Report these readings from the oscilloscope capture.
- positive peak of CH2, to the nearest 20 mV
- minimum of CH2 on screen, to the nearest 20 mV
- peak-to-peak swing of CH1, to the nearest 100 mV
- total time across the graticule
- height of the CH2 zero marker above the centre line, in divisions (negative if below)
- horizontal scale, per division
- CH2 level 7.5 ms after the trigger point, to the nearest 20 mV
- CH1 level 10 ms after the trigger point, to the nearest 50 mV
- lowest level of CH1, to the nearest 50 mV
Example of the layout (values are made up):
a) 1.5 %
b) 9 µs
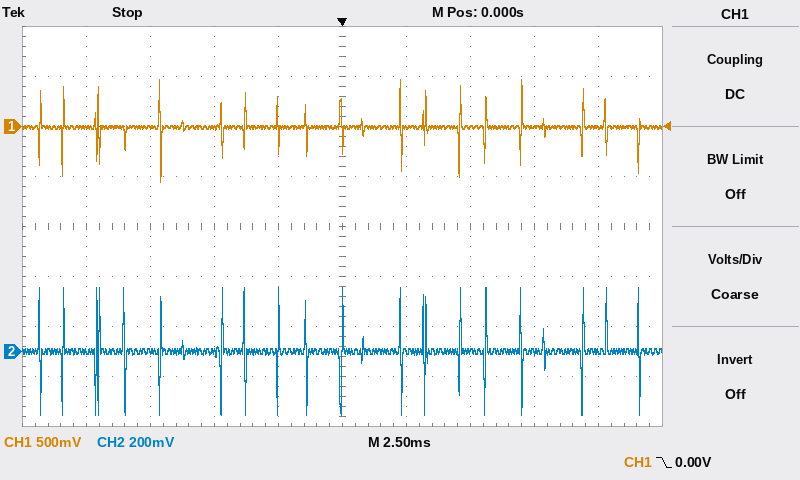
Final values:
a) 260 mV
b) -260 mV
c) 1.00 V
d) 25 ms
e) -2.5 div
f) 2.5 ms
g) 0 mV
h) 0 mV
i) -550 mV
